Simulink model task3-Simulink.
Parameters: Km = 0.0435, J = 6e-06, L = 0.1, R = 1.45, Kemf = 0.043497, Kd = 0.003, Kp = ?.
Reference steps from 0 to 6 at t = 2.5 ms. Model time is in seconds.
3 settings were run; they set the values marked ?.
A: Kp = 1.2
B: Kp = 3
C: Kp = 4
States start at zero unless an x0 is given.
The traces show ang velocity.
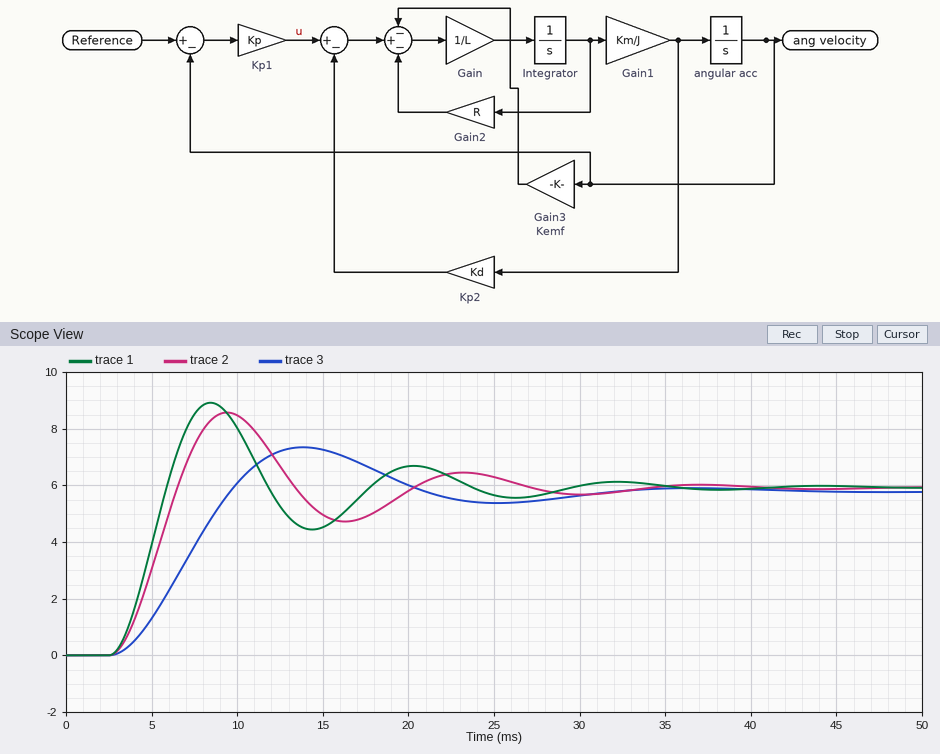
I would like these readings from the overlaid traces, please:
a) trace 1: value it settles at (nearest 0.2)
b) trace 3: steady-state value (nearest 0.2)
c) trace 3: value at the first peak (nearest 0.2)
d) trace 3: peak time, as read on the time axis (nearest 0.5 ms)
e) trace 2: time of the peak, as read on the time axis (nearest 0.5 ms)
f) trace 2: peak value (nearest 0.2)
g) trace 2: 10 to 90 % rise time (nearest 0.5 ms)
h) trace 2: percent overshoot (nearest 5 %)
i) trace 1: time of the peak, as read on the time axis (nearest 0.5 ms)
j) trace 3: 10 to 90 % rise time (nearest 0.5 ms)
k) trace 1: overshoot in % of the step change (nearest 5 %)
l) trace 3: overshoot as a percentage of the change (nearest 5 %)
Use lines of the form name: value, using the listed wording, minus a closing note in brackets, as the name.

trace 1: value it settles at: 6.0
trace 3: steady-state value: 5.8
trace 3: value at the first peak: 7.4
trace 3: peak time, as read on the time axis: 14.0 ms
trace 2: time of the peak, as read on the time axis: 9.5 ms
trace 2: peak value: 8.6
trace 2: 10 to 90 % rise time: 2.5 ms
trace 2: percent overshoot: 45 %
trace 1: time of the peak, as read on the time axis: 8.5 ms
trace 3: 10 to 90 % rise time: 5.0 ms
trace 1: overshoot in % of the step change: 50 %
trace 3: overshoot as a percentage of the change: 25 %
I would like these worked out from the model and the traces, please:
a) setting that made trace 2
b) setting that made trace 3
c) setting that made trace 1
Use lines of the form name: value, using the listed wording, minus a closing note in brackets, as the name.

setting that made trace 2: B
setting that made trace 3: A
setting that made trace 1: C
